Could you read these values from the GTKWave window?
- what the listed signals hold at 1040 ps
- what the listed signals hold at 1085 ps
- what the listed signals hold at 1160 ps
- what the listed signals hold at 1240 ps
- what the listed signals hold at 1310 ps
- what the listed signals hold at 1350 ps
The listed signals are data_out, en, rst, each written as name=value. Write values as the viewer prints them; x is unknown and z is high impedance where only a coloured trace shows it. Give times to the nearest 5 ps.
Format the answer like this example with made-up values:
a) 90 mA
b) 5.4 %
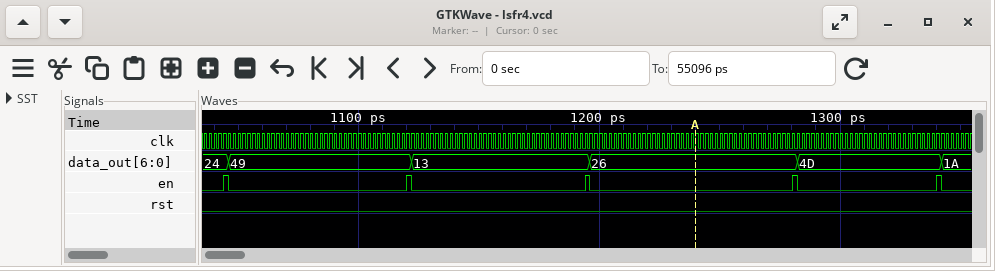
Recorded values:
a) data_out=24, en=0, rst=0
b) data_out=49, en=0, rst=0
c) data_out=13, en=0, rst=0
d) data_out=26, en=0, rst=0
e) data_out=4D, en=0, rst=0
f) data_out=1A, en=0, rst=0
